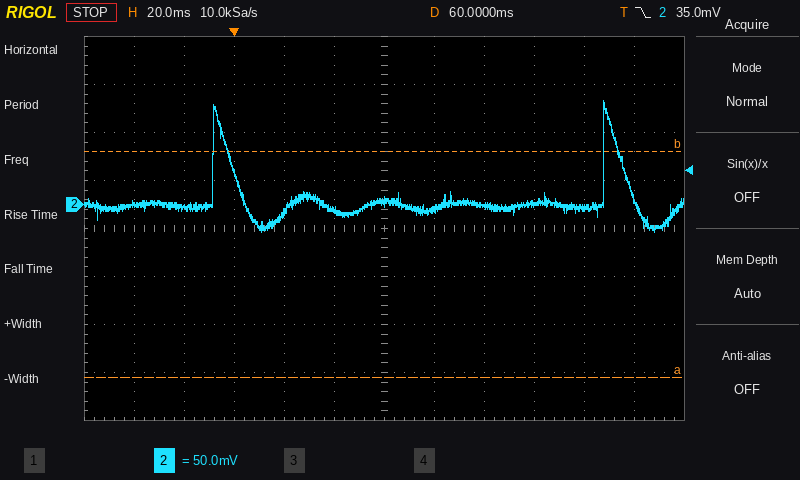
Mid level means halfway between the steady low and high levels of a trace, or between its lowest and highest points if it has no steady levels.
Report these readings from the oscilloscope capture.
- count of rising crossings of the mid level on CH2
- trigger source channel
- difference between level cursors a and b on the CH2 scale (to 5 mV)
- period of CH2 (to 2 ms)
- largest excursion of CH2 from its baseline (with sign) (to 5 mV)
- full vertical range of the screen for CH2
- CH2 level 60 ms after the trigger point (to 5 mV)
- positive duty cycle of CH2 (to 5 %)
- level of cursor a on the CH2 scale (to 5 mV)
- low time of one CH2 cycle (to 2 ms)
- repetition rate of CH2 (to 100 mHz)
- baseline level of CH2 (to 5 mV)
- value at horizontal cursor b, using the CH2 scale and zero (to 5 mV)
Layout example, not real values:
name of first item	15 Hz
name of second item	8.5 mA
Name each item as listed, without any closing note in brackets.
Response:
count of rising crossings of the mid level on CH2	2
trigger source channel	CH2
difference between level cursors a and b on the CH2 scale	235 mV
period of CH2	156 ms
largest excursion of CH2 from its baseline (with sign)	+110 mV
full vertical range of the screen for CH2	400 mV
CH2 level 60 ms after the trigger point	5 mV
positive duty cycle of CH2	5 %
level of cursor a on the CH2 scale	-180 mV
low time of one CH2 cycle	148 ms
repetition rate of CH2	6.4 Hz
baseline level of CH2	0 mV
value at horizontal cursor b, using the CH2 scale and zero	55 mV
